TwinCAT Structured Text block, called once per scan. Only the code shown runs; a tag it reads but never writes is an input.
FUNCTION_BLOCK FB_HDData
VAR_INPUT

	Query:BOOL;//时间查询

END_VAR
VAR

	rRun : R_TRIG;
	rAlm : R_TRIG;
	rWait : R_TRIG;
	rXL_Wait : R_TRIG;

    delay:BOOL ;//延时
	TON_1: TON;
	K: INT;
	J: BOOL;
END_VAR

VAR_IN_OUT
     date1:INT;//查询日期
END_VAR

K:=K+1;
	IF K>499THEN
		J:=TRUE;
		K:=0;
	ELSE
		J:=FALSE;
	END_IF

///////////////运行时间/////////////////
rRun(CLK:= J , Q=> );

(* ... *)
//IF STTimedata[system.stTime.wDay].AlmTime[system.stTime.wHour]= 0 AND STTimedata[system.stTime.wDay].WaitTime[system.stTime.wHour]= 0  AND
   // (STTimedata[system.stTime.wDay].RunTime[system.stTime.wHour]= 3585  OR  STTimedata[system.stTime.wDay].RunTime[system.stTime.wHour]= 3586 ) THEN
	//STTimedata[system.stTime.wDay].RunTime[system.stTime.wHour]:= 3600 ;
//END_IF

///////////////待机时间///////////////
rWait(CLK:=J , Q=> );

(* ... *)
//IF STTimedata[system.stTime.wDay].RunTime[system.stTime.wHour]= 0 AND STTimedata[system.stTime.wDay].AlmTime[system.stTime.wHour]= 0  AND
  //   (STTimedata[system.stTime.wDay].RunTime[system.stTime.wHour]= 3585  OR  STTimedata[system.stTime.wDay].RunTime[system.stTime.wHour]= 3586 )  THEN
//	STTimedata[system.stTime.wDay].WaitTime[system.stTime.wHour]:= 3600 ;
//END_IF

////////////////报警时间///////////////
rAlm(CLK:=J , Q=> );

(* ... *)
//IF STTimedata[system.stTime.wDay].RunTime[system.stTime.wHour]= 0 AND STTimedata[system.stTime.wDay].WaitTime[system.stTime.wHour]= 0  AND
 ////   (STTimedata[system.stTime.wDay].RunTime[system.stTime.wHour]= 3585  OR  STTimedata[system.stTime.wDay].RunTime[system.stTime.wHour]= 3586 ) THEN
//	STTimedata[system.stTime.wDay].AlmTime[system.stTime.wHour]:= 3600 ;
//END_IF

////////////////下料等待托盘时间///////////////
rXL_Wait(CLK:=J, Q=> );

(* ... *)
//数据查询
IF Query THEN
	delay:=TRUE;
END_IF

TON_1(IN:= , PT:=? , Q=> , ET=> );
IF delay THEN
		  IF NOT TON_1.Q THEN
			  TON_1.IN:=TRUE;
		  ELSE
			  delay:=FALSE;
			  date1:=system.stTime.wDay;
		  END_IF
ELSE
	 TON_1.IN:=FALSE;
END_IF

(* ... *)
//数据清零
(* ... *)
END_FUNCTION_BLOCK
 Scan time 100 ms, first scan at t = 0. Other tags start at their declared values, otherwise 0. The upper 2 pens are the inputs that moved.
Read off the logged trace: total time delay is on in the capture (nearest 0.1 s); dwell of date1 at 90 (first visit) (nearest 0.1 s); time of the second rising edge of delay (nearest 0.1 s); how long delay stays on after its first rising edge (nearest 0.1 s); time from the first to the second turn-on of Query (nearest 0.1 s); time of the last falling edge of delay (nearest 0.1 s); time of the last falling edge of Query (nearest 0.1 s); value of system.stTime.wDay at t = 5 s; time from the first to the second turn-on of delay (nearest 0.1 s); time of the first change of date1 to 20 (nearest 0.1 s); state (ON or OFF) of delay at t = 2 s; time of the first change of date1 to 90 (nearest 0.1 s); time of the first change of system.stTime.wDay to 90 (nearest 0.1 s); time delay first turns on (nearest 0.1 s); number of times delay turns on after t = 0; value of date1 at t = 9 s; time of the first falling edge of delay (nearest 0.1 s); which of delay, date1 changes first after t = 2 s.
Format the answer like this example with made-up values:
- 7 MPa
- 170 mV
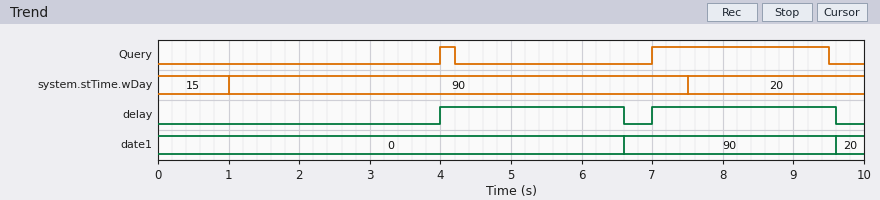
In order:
- 5.2 s
- 3.0 s
- 7.0 s
- 2.6 s
- 3.0 s
- 9.6 s
- 9.5 s
- 90
- 3.0 s
- 9.6 s
- OFF
- 6.6 s
- 1.0 s
- 4.0 s
- 2
- 90
- 6.6 s
- delay
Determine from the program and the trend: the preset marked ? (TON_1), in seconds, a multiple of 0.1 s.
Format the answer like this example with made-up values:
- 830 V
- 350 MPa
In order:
- 2.5 s
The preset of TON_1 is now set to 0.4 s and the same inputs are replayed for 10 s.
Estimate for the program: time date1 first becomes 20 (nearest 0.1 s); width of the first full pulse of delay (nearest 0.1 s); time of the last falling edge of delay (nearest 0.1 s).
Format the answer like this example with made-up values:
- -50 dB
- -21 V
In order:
- 7.5 s
- 0.5 s
- 7.5 s
